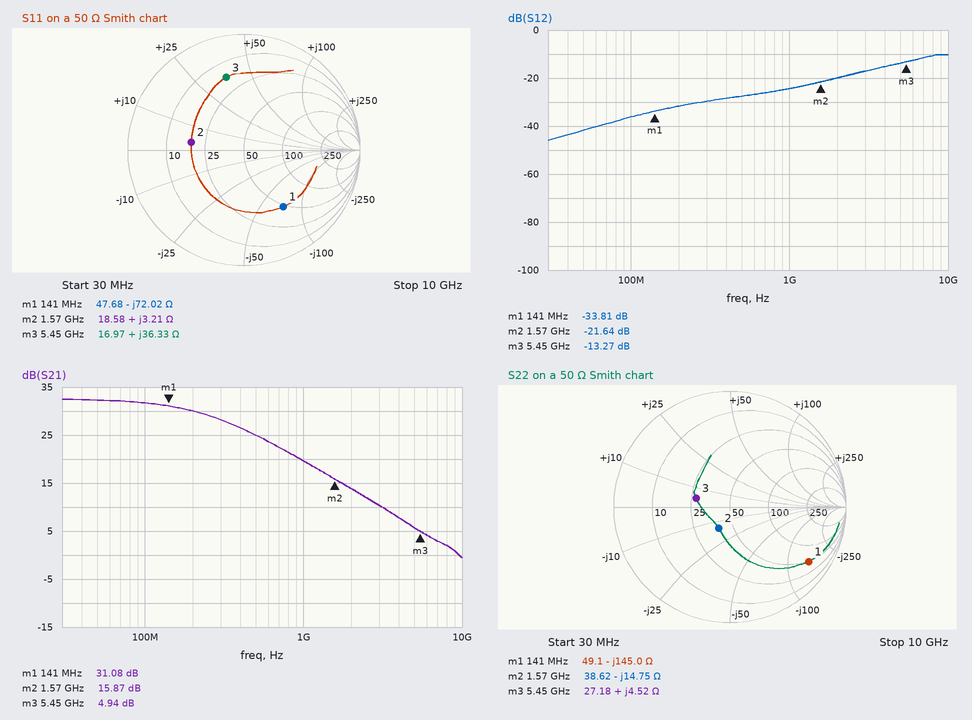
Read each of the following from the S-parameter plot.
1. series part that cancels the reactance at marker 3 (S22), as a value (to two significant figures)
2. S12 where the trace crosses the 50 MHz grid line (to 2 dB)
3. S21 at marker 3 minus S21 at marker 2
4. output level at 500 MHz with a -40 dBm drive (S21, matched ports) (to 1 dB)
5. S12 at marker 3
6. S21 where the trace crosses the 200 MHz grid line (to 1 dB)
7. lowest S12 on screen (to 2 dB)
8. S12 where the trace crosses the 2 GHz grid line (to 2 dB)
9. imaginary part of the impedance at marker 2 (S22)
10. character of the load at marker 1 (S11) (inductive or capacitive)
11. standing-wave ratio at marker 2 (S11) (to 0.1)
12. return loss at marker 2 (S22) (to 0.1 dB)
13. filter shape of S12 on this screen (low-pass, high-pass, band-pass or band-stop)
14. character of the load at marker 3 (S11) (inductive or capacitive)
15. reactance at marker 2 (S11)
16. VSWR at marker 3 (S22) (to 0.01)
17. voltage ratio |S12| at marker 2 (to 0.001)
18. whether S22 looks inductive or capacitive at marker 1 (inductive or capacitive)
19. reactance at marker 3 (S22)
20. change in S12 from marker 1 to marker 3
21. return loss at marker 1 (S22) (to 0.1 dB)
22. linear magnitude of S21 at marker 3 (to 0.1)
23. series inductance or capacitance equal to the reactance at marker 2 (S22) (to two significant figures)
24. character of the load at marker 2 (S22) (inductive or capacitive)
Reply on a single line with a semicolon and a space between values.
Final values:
6.5 pF; -42 dB; -10.93 dB; -15 dBm; -13.27 dB; 30 dB; -46 dB; -20 dB; -14.75 Ω; capacitive; 2.7; 13.7 dB; high-pass; inductive; +3.21 Ω; 1.86; 0.083; capacitive; +4.52 Ω; 20.54 dB; 1.7 dB; 1.8; 6.9 pF; capacitive
